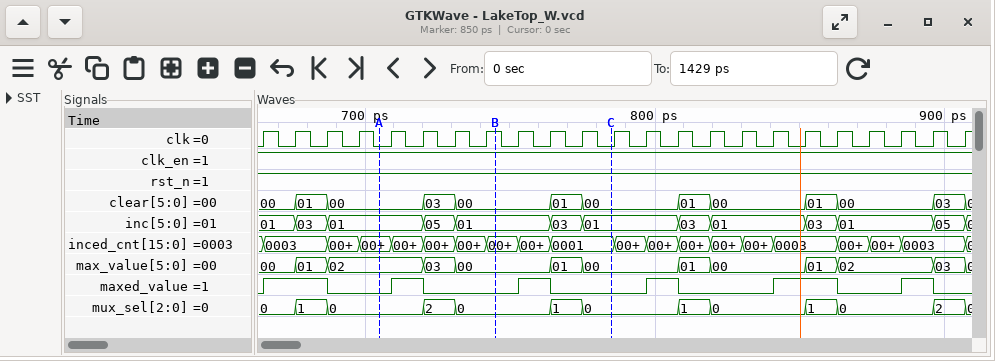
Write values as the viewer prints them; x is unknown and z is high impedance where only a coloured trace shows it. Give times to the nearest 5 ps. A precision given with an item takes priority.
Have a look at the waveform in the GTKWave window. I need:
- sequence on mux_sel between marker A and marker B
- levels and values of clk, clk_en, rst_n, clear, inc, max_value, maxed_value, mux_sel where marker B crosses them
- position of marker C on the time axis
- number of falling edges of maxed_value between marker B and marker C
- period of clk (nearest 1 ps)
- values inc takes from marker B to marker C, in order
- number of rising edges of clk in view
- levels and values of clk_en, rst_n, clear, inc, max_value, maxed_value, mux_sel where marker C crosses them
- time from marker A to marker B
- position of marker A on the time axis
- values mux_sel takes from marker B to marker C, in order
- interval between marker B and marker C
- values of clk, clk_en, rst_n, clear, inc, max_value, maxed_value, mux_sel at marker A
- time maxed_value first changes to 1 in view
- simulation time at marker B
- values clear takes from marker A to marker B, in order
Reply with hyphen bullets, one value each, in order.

- 0, 2, 0
- clk=1, clk_en=1, rst_n=1, clear=00, inc=01, max_value=00, maxed_value=0, mux_sel=0
- 785 ps
- 1
- 11 ps
- 01, 03, 01
- 23
- clk_en=1, rst_n=1, clear=00, inc=01, max_value=00, maxed_value=0, mux_sel=0
- 40 ps
- 705 ps
- 0, 1, 0
- 40 ps
- clk=0, clk_en=1, rst_n=1, clear=00, inc=01, max_value=02, maxed_value=0, mux_sel=0
- 665 ps
- 745 ps
- 00, 03, 00
